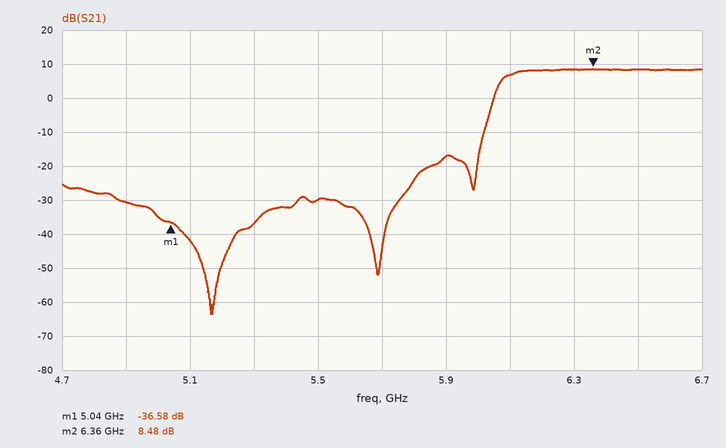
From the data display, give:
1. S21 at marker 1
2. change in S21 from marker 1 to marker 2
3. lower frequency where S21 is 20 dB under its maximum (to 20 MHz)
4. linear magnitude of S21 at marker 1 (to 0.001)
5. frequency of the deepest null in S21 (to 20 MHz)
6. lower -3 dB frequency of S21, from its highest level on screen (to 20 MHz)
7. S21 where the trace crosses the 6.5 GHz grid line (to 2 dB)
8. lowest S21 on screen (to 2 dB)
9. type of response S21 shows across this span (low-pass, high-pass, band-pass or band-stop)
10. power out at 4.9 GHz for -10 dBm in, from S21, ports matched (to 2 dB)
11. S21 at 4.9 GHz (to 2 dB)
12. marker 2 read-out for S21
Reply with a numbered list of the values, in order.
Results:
1. -36.58 dB
2. 45.06 dB
3. 6.02 GHz
4. 0.015
5. 5.16 GHz
6. 6.08 GHz
7. 8 dB
8. -64 dB
9. high-pass
10. -40 dBm
11. -30 dB
12. 8.48 dB
